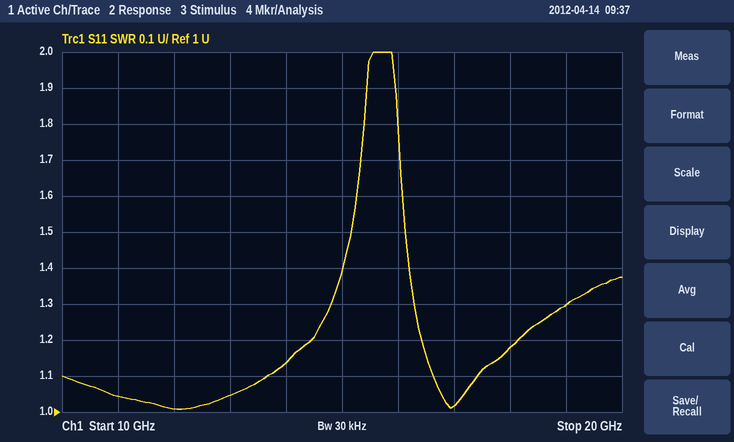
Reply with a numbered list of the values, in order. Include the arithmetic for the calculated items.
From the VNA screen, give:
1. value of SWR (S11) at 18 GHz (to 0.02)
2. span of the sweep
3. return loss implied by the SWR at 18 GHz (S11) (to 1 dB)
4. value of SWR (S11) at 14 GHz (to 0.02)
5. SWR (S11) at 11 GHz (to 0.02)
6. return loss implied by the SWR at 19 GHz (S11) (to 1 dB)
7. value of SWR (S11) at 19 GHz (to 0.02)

1. 1.18
2. 10 GHz
3. −20 log10((1.18 − 1)/(1.18 + 1)) ≈ 22 dB
4. 1.14
5. 1.04
6. −20 log10((1.3 − 1)/(1.3 + 1)) ≈ 18 dB
7. 1.30
